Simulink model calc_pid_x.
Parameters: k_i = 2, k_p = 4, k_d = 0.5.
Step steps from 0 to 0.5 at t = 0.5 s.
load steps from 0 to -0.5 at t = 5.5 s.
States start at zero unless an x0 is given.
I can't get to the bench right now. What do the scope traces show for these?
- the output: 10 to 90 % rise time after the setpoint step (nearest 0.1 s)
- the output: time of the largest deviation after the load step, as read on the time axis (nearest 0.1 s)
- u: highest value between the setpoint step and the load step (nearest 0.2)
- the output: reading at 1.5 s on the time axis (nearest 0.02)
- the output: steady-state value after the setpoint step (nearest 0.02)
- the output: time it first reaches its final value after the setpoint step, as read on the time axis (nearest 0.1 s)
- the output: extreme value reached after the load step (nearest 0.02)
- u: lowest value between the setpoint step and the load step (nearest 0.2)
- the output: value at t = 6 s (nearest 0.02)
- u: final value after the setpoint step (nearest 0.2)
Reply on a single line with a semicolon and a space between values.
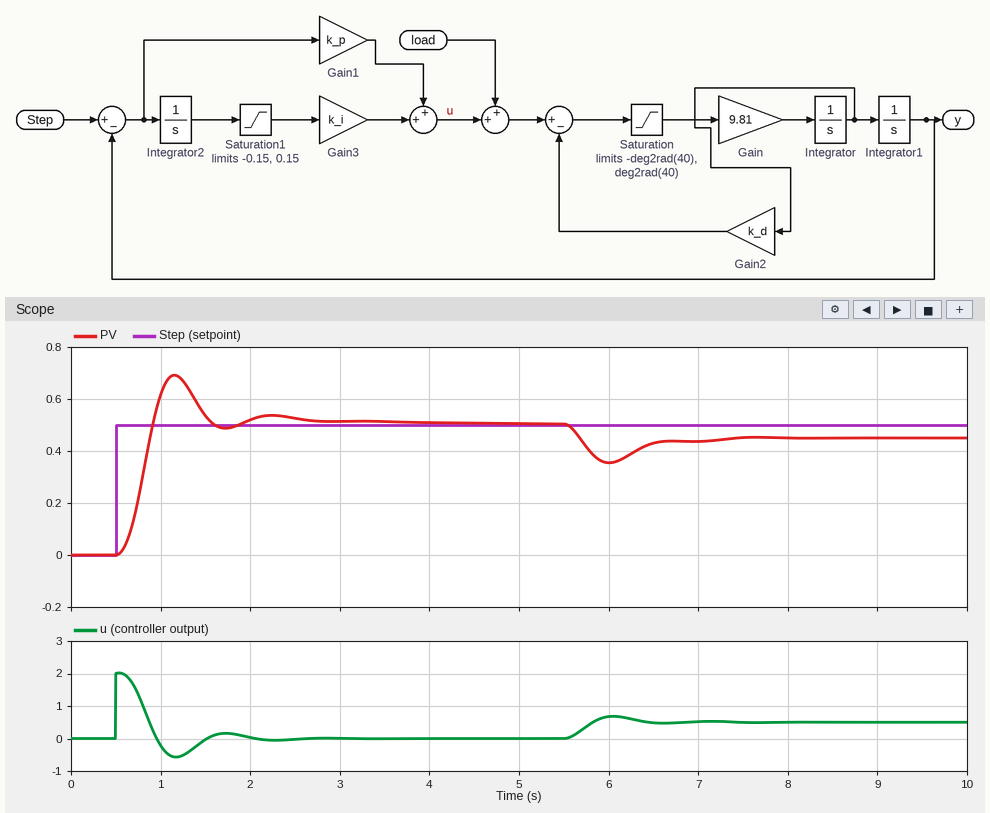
0.3 s; 6.0 s; 2.0; 0.54; 0.50; 0.9 s; 0.36; -0.6; 0.36; 0.0
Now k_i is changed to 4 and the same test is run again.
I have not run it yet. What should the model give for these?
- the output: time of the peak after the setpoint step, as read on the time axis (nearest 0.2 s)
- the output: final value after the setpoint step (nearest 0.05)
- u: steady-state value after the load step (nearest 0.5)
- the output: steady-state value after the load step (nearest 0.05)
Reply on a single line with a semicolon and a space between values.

1.2 s; 0.50; 0.5; 0.50
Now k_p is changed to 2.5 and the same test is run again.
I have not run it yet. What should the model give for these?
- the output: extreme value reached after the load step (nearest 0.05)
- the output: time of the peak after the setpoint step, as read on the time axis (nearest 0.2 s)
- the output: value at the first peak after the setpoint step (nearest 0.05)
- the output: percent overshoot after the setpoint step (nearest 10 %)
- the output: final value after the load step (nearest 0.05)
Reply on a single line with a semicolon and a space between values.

0.30; 1.2 s; 0.70; 40 %; 0.40
